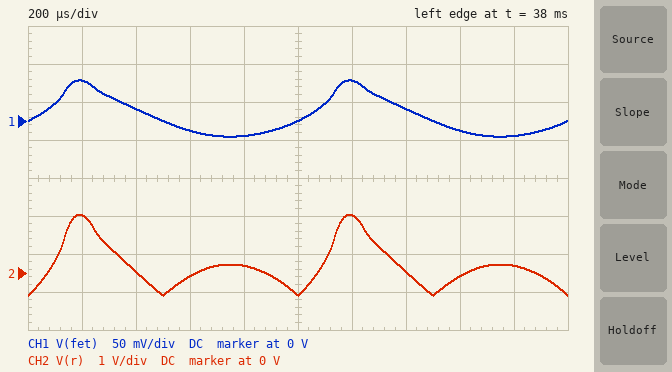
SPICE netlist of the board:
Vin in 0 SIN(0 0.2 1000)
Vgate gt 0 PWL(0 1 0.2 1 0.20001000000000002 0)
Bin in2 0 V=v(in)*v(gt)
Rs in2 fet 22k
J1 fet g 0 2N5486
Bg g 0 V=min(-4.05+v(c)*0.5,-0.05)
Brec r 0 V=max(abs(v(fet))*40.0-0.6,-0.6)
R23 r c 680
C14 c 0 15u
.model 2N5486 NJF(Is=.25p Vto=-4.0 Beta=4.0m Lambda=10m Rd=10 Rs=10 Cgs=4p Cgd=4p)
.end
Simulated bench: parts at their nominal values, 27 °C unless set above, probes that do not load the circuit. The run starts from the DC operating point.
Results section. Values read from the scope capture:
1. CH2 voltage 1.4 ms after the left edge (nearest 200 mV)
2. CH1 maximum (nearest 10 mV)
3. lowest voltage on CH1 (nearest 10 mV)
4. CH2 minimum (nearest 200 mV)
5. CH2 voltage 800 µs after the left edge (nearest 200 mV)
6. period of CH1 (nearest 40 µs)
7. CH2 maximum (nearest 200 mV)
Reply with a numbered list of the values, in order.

1. 0 V
2. 50 mV
3. -20 mV
4. -600 mV
5. 200 mV
6. 1.00 ms
7. 1.6 V
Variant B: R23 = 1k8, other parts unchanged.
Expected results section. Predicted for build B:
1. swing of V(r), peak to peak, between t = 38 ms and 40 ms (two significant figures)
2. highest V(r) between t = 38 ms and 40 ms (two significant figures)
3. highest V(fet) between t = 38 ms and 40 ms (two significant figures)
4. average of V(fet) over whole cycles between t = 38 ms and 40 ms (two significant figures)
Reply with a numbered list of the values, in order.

1. 2.2 V
2. 1.6 V
3. 55 mV
4. 6.1 mV
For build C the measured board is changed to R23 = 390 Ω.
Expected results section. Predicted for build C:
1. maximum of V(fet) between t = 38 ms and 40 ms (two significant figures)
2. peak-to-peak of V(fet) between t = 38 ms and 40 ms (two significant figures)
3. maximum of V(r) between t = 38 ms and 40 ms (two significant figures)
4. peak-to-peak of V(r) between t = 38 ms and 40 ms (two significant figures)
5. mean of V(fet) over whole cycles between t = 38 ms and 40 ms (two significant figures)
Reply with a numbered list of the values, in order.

1. 51 mV
2. 72 mV
3. 1.4 V
4. 2.0 V
5. 5.5 mV
